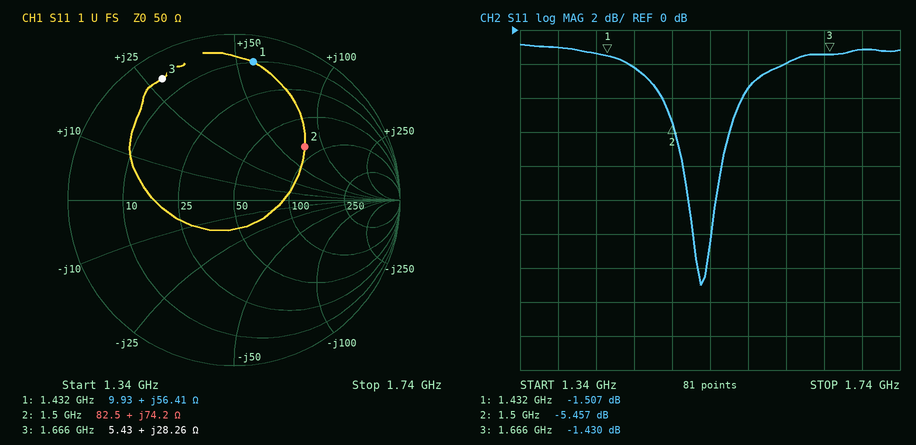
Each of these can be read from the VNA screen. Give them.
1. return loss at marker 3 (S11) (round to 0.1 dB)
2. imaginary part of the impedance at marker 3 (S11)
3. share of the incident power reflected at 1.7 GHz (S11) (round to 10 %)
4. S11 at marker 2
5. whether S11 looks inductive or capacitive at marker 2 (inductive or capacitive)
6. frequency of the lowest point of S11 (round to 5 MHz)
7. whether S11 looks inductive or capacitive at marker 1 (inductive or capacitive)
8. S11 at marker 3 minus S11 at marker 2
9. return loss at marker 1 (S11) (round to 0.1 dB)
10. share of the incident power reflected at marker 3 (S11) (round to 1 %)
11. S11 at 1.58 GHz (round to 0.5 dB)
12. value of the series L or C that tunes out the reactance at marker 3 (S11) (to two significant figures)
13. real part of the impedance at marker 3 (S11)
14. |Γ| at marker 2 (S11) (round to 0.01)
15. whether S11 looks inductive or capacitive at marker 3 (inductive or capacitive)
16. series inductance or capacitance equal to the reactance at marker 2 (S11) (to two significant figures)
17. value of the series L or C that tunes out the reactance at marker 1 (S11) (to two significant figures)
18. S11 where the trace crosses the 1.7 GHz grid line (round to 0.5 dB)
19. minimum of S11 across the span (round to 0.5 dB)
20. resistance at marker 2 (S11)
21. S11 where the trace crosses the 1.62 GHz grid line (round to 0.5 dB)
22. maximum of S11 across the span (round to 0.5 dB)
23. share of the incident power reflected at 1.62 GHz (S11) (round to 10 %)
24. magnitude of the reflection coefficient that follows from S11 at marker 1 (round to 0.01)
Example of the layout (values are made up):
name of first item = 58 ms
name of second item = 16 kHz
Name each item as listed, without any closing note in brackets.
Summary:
return loss at marker 3 (S11) = 1.4 dB
imaginary part of the impedance at marker 3 = +28.26 Ω
share of the incident power reflected at 1.7 GHz (S11) = 80 %
S11 at marker 2 = -5.457 dB
whether S11 looks inductive or capacitive at marker 2 = inductive
frequency of the lowest point of S11 = 1.530 GHz
whether S11 looks inductive or capacitive at marker 1 = inductive
S11 at marker 3 minus S11 at marker 2 = 4.027 dB
return loss at marker 1 (S11) = 1.5 dB
share of the incident power reflected at marker 3 (S11) = 72 %
S11 at 1.58 GHz = -3.5 dB
value of the series L or C that tunes out the reactance at marker 3 (S11) = 3.4 pF
real part of the impedance at marker 3 = 5.43 Ω
|Γ| at marker 2 (S11) = 0.53
whether S11 looks inductive or capacitive at marker 3 = inductive
series inductance or capacitance equal to the reactance at marker 2 (S11) = 7.9 nH
value of the series L or C that tunes out the reactance at marker 1 (S11) = 2.0 pF
S11 where the trace crosses the 1.7 GHz grid line = -1.0 dB
minimum of S11 across the span = -15.0 dB
resistance at marker 2 = 82.5 Ω
S11 where the trace crosses the 1.62 GHz grid line = -2.0 dB
maximum of S11 across the span = -1.0 dB
share of the incident power reflected at 1.62 GHz (S11) = 60 %
magnitude of the reflection coefficient that follows from S11 at marker 1 = 0.84
